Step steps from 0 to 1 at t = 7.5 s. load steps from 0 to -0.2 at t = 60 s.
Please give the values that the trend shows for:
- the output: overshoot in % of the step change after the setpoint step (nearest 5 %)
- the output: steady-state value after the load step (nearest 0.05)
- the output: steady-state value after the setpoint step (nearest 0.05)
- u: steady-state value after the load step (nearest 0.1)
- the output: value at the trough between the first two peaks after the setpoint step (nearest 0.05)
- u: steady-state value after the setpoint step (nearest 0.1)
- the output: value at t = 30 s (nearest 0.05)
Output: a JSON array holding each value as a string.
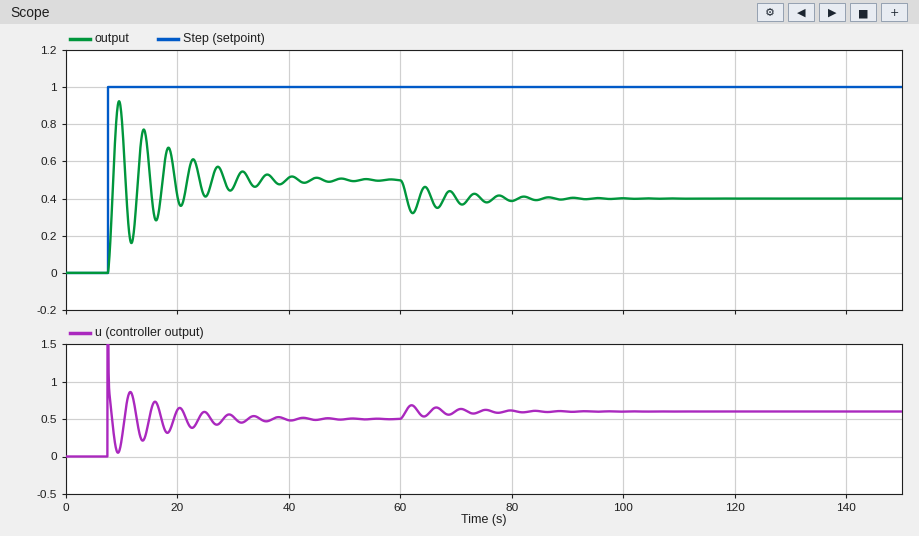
["85 %", "0.40", "0.50", "0.6", "0.15", "0.5", "0.45"]
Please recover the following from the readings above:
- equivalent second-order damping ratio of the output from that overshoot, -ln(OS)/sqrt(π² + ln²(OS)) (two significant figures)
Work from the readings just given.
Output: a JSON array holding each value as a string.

["0.052"]
